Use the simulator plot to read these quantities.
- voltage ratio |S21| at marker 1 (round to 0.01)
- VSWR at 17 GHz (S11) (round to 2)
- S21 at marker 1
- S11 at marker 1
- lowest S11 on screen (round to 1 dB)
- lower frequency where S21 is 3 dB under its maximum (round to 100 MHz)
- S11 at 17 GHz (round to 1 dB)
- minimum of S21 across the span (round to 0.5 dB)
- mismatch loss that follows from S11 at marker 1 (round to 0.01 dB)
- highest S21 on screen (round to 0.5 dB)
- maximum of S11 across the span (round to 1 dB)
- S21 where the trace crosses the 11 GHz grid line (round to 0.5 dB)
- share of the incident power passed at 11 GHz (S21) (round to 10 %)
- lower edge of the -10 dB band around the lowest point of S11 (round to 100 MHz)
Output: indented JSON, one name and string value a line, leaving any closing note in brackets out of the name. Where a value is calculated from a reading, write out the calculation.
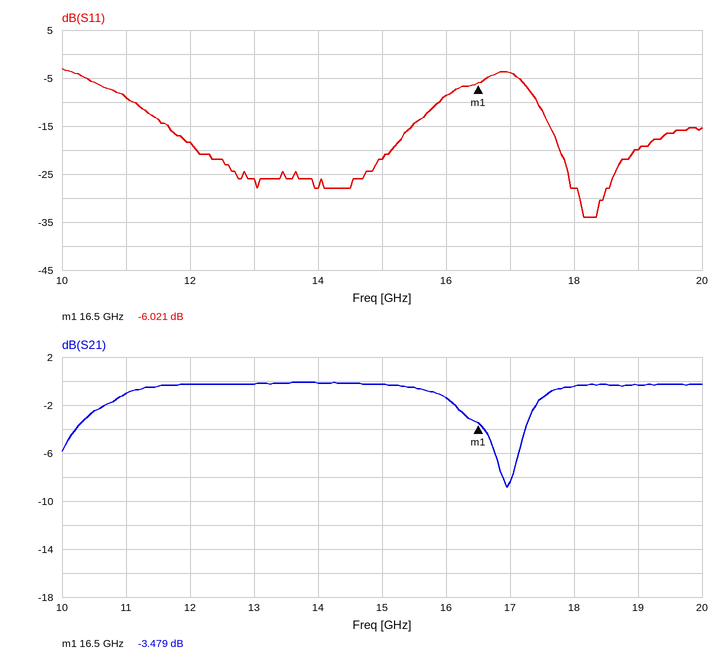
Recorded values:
{
  "voltage ratio |S21| at marker 1": "10^(-3.479/20) ≈ 0.67",
  "VSWR at 17 GHz (S11)": "|Γ| = 10^(-4/20) = 0.6310; VSWR = (1 + 0.6310)/(1 − 0.6310) ≈ 4",
  "S21 at marker 1": "-3.479 dB",
  "S11 at marker 1": "-6.021 dB",
  "lowest S11 on screen": "-34 dB",
  "lower frequency where S21 is 3 dB under its maximum": "10.4 GHz",
  "S11 at 17 GHz": "-4 dB",
  "minimum of S21 across the span": "-9.0 dB",
  "mismatch loss that follows from S11 at marker 1": "−10 log10(1 − 10^(-6.021/10)) ≈ 1.25 dB",
  "highest S21 on screen": "0.0 dB",
  "maximum of S11 across the span": "-3 dB",
  "S21 where the trace crosses the 11 GHz grid line": "-1.0 dB",
  "share of the incident power passed at 11 GHz (S21)": "10^(-1/10) ≈ 79.4 %, so 80 % to the nearest 10 %",
  "lower edge of the -10 dB band around the lowest point of S11": "17.4 GHz"
}
